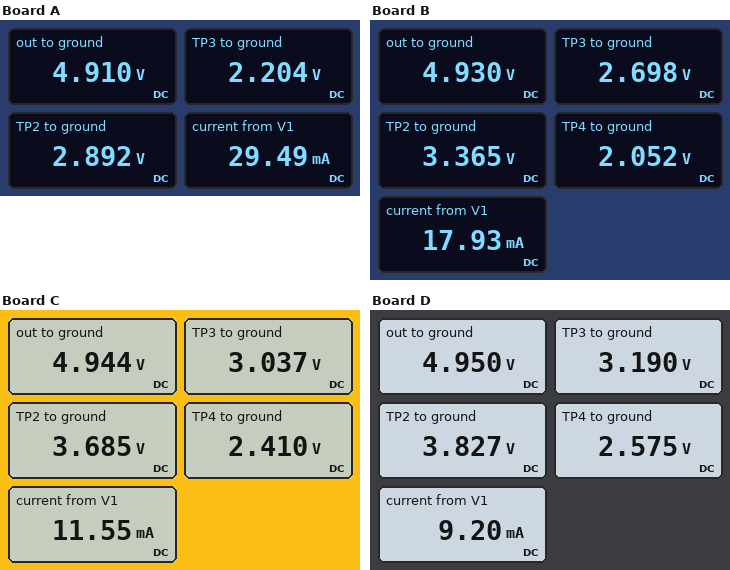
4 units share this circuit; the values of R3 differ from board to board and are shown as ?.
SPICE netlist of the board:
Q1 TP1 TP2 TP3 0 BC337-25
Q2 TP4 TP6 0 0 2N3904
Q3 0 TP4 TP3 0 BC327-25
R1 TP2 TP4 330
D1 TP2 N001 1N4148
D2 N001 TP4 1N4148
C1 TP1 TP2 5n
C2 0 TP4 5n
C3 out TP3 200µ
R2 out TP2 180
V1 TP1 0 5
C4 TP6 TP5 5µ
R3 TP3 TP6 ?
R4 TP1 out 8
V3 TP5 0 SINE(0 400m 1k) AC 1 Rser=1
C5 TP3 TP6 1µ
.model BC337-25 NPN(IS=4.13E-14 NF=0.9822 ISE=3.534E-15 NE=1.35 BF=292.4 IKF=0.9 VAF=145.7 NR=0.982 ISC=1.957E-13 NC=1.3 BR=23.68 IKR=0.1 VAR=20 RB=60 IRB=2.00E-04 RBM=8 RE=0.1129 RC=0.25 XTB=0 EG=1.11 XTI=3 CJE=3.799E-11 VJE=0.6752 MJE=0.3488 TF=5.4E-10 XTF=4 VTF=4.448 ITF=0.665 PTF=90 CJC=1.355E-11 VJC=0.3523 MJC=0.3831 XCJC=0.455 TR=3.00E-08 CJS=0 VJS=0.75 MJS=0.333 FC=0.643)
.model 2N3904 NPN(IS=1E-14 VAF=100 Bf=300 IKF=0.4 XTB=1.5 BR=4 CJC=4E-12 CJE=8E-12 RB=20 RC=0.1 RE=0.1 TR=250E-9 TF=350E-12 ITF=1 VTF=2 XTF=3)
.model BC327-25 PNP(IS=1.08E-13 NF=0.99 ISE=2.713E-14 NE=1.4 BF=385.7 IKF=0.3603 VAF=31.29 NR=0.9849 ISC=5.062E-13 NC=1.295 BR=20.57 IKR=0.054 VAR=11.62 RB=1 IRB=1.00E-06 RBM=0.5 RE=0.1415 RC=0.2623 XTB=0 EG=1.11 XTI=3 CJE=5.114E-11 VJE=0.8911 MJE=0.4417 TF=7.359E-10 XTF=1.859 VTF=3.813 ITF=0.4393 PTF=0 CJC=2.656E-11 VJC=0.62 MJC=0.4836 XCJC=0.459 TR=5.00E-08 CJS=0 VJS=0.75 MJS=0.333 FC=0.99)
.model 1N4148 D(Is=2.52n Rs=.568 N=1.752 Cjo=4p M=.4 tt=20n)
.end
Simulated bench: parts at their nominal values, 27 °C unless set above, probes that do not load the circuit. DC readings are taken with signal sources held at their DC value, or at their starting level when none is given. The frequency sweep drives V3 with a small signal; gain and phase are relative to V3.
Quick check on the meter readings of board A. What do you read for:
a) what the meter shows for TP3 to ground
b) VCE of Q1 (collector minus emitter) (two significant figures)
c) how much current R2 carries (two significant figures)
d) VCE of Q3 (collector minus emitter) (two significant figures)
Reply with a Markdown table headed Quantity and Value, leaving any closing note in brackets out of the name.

| Quantity | Value |
|---|---|
| what the meter shows for TP3 to ground | 2.204 V |
| VCE of Q1 (collector minus emitter) | 2.8 V |
| how much current R2 carries | 11 mA |
| VCE of Q3 (collector minus emitter) | -2.2 V |
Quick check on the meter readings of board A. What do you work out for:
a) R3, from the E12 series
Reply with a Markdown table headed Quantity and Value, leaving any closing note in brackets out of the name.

| Quantity | Value |
|---|---|
| R3, from the E12 series | 39 kΩ |
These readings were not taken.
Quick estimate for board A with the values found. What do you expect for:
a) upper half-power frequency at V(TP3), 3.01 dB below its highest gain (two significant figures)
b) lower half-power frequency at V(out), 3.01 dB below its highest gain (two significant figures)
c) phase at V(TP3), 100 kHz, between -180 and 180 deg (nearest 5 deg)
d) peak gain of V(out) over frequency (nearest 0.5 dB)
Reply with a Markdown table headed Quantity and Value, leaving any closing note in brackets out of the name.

| Quantity | Value |
|---|---|
| upper half-power frequency at V(TP3), 3.01 dB below its highest gain | 31 kHz |
| lower half-power frequency at V(out), 3.01 dB below its highest gain | 110 Hz |
| phase at V(TP3), 100 kHz, between -180 and 180 deg | 105 deg |
| peak gain of V(out) over frequency | 14.0 dB |
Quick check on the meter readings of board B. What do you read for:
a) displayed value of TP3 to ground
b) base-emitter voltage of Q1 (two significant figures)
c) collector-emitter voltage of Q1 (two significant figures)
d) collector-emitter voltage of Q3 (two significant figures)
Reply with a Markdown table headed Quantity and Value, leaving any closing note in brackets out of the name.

| Quantity | Value |
|---|---|
| displayed value of TP3 to ground | 2.698 V |
| base-emitter voltage of Q1 | 670 mV |
| collector-emitter voltage of Q1 | 2.3 V |
| collector-emitter voltage of Q3 | -2.7 V |
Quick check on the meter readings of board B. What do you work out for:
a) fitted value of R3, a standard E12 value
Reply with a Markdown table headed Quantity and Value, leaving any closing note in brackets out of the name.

| Quantity | Value |
|---|---|
| fitted value of R3, a standard E12 value | 68 kΩ |
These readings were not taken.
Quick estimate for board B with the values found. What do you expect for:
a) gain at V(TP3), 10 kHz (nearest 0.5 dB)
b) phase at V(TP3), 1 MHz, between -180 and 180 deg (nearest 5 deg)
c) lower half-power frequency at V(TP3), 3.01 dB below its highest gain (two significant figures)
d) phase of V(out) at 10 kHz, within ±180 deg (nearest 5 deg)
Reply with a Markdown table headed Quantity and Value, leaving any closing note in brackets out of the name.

| Quantity | Value |
|---|---|
| gain at V(TP3), 10 kHz | 13.5 dB |
| phase at V(TP3), 1 MHz, between -180 and 180 deg | 60 deg |
| lower half-power frequency at V(TP3), 3.01 dB below its highest gain | 5.3 Hz |
| phase of V(out) at 10 kHz, within ±180 deg | 160 deg |
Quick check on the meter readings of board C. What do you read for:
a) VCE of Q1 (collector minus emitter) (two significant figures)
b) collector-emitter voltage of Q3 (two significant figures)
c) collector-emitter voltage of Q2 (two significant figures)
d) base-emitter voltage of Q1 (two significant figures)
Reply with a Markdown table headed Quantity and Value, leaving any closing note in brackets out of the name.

| Quantity | Value |
|---|---|
| VCE of Q1 (collector minus emitter) | 2.0 V |
| collector-emitter voltage of Q3 | -3.0 V |
| collector-emitter voltage of Q2 | 2.4 V |
| base-emitter voltage of Q1 | 650 mV |
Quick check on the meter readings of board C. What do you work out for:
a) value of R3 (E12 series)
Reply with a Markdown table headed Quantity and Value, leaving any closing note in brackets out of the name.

| Quantity | Value |
|---|---|
| value of R3 | 100 kΩ |
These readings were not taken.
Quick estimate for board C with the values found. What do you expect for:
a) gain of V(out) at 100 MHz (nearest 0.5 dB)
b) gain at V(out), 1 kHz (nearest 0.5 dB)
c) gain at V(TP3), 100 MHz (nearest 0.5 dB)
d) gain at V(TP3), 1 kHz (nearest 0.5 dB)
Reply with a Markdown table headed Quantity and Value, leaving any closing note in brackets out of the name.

| Quantity | Value |
|---|---|
| gain of V(out) at 100 MHz | -2.5 dB |
| gain at V(out), 1 kHz | 13.5 dB |
| gain at V(TP3), 100 MHz | -2.5 dB |
| gain at V(TP3), 1 kHz | 13.5 dB |
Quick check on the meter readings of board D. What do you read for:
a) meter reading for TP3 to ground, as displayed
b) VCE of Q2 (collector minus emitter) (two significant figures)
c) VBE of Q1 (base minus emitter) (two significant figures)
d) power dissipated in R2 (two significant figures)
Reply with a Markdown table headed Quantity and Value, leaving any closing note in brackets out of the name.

| Quantity | Value |
|---|---|
| meter reading for TP3 to ground, as displayed | 3.190 V |
| VCE of Q2 (collector minus emitter) | 2.6 V |
| VBE of Q1 (base minus emitter) | 640 mV |
| power dissipated in R2 | 7.0 mW |
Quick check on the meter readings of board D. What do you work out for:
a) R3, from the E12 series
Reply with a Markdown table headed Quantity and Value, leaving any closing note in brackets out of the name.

| Quantity | Value |
|---|---|
| R3, from the E12 series | 120 kΩ |
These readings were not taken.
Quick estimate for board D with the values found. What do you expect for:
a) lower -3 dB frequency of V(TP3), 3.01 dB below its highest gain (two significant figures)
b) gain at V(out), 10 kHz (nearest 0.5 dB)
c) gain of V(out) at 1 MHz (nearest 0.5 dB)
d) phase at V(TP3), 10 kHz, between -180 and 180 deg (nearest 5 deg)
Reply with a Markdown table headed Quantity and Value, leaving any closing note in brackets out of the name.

| Quantity | Value |
|---|---|
| lower -3 dB frequency of V(TP3), 3.01 dB below its highest gain | 3.8 Hz |
| gain at V(out), 10 kHz | 13.0 dB |
| gain of V(out) at 1 MHz | -3.0 dB |
| phase at V(TP3), 10 kHz, between -180 and 180 deg | 160 deg |
